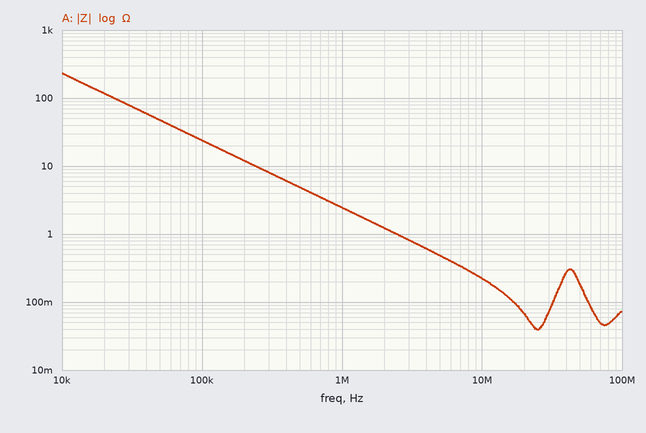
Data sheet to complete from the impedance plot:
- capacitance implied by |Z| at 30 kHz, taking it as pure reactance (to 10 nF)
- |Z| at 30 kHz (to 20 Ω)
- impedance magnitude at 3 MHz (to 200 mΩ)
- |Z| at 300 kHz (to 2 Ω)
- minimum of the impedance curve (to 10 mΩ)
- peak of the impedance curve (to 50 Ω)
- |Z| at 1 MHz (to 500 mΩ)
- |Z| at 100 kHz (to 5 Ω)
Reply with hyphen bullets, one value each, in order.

- 70 nF
- 80 Ω
- 800 mΩ
- 8 Ω
- 40 mΩ
- 250 Ω
- 2.5 Ω
- 25 Ω
